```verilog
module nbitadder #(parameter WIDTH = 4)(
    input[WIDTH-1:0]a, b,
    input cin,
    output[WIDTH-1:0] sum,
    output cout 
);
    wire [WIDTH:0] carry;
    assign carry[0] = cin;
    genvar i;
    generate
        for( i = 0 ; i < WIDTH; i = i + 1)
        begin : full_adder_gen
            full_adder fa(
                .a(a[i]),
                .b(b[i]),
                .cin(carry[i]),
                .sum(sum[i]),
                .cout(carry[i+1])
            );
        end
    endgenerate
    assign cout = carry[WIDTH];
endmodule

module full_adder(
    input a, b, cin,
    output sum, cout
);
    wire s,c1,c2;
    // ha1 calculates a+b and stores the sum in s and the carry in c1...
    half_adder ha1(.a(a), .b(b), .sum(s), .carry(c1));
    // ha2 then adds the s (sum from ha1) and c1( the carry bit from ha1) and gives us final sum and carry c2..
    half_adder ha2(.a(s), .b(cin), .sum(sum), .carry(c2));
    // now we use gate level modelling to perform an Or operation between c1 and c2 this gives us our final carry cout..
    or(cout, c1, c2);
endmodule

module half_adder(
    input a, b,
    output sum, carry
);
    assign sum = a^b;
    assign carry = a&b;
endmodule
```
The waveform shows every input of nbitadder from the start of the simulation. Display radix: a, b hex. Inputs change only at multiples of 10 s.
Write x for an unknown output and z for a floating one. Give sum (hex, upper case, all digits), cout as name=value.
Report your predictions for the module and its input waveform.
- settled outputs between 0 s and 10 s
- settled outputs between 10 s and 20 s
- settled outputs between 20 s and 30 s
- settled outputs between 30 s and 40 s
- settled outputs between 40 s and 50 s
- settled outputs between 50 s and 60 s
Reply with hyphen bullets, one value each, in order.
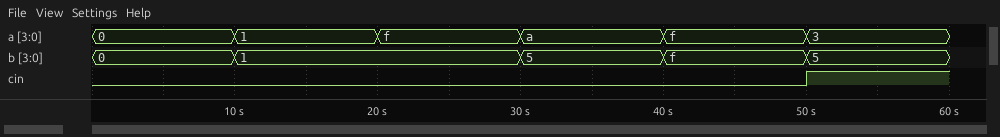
- sum=0, cout=0
- sum=2, cout=0
- sum=0, cout=1
- sum=F, cout=0
- sum=E, cout=1
- sum=9, cout=0
